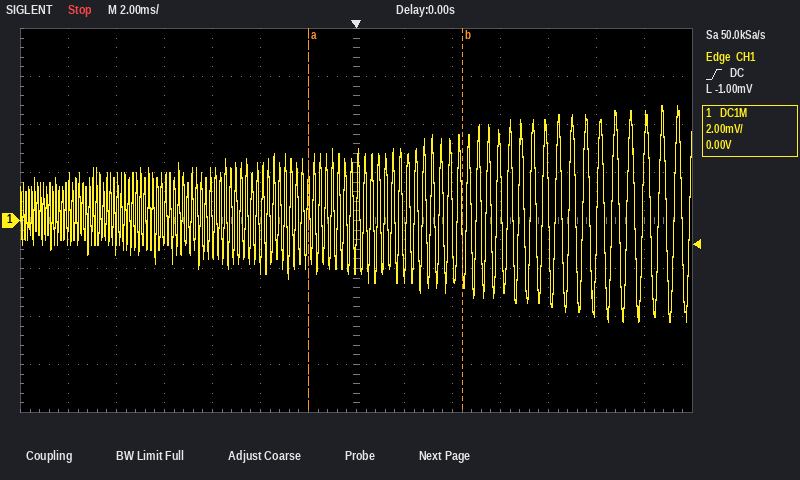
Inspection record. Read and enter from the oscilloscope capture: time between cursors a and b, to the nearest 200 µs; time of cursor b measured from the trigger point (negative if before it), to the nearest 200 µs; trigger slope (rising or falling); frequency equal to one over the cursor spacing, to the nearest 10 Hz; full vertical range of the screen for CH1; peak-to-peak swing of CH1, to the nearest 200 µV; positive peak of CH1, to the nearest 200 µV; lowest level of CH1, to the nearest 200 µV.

6.4 ms
+4.4 ms
rising
160 Hz
16 mV
9.0 mV
4.8 mV
-4.2 mV
